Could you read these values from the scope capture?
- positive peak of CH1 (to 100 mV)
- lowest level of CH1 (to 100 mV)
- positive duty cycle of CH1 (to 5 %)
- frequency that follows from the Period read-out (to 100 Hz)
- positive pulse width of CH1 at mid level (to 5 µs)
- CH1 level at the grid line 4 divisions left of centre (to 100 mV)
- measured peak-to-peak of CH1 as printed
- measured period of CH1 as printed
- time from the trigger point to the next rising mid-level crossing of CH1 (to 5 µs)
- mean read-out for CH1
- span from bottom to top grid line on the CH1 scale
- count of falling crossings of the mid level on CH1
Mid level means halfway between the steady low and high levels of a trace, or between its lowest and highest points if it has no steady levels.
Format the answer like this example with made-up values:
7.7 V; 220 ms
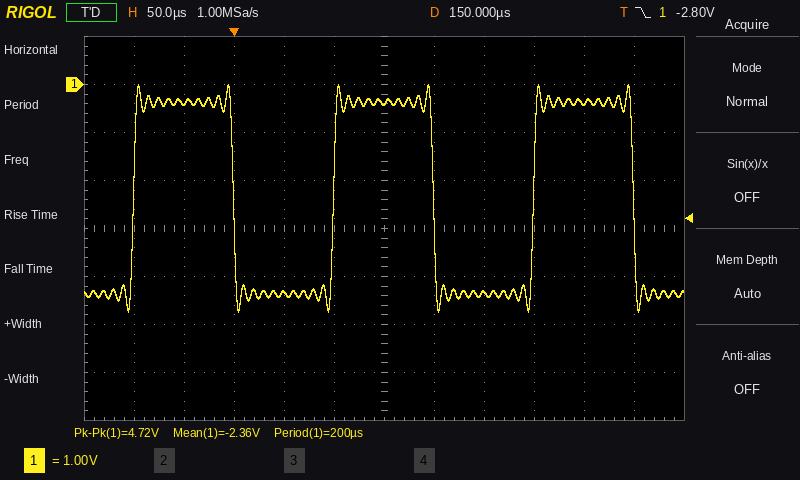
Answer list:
0.0 V; -4.7 V; 50 %; 5.0 kHz; 100 µs; -400 mV; 4.72 V; 200 µs; 100 µs; -2.36 V; 8 V; 3
